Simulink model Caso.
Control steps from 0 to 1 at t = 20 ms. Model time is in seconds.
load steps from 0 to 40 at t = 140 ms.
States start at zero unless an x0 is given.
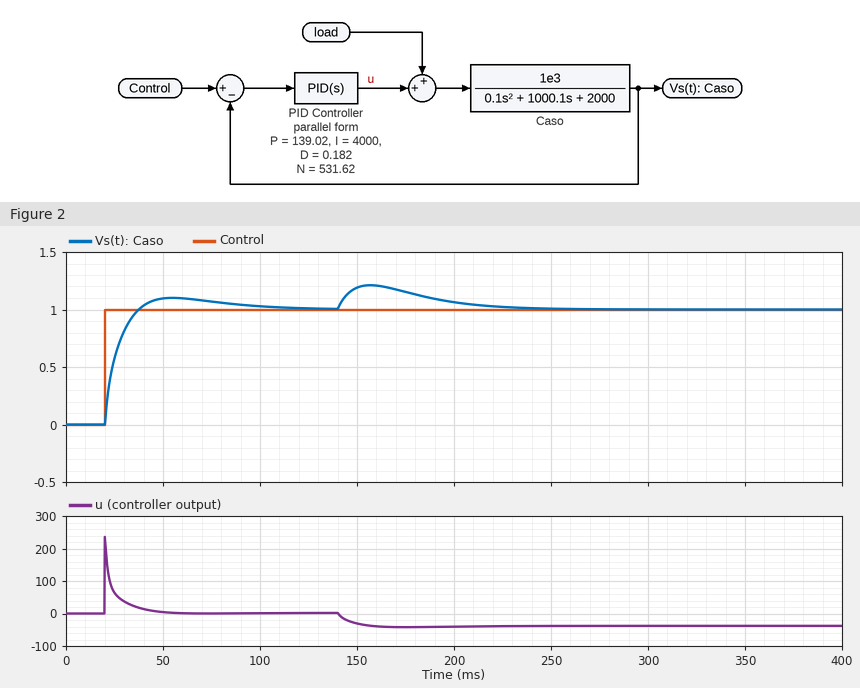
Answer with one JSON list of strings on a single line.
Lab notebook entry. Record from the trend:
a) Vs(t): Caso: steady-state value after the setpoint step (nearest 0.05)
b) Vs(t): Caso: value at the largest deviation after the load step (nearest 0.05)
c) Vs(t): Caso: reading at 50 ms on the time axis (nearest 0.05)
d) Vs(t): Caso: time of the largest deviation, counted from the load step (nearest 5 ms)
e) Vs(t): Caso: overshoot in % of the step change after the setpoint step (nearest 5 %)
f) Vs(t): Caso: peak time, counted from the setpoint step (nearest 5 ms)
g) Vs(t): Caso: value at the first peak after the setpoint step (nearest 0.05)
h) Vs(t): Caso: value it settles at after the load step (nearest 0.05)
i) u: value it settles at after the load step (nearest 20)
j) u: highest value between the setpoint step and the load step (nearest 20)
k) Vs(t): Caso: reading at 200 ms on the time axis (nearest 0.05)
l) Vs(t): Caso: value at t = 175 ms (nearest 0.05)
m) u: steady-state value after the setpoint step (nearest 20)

["1.00", "1.20", "1.10", "15 ms", "10 %", "35 ms", "1.10", "1.00", "-40", "240", "1.05", "1.15", "0"]
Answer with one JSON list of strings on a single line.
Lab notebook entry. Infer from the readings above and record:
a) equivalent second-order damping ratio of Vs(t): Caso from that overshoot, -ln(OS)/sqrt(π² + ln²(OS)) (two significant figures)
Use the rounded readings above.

["0.59"]
